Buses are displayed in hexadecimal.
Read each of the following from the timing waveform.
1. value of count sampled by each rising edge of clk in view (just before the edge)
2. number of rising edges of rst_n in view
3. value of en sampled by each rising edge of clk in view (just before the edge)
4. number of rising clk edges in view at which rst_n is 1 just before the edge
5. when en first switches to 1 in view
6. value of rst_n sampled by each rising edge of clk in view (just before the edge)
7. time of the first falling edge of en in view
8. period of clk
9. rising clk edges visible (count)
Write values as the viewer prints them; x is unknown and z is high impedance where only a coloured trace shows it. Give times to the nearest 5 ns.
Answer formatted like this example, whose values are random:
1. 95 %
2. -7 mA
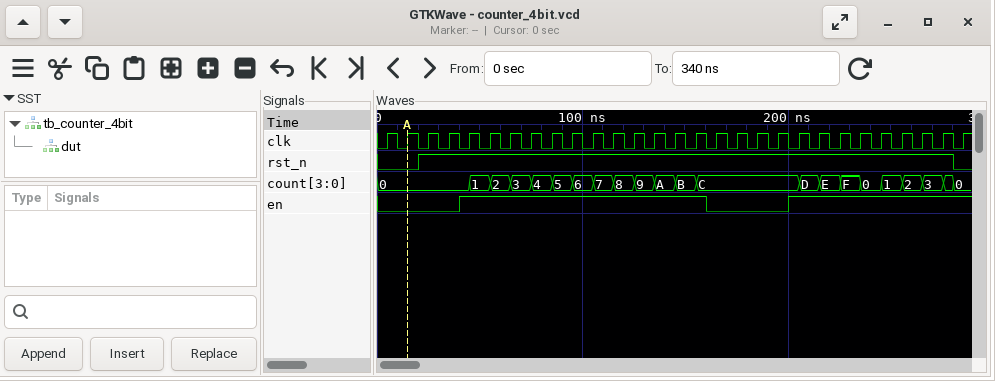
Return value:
1. 0, 0, 0, 0, 0, 1, 2, 3, 4, 5, 6, 7, 8, 9, A, B, C, C, C, C, C, D, E, F, 0, 1, 2, 3, 0
2. 1
3. 0 0 0 0 1 1 1 1 1 1 1 1 1 1 1 1 0 0 0 0 1 1 1 1 1 1 1 1 1
4. 26
5. 40 ns
6. 0 0 1 1 1 1 1 1 1 1 1 1 1 1 1 1 1 1 1 1 1 1 1 1 1 1 1 1 0
7. 160 ns
8. 10 ns
9. 29
